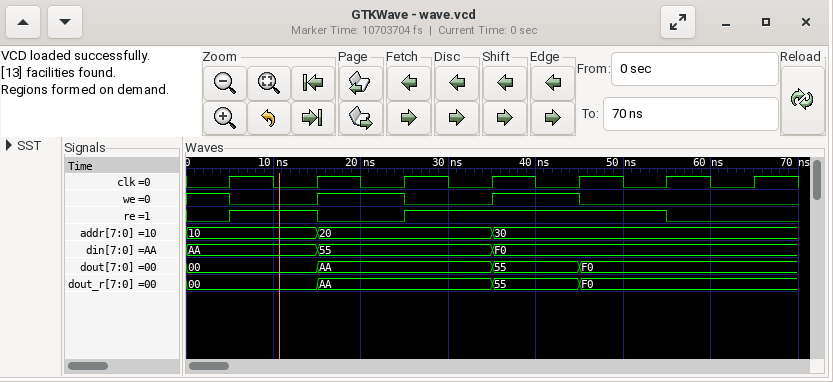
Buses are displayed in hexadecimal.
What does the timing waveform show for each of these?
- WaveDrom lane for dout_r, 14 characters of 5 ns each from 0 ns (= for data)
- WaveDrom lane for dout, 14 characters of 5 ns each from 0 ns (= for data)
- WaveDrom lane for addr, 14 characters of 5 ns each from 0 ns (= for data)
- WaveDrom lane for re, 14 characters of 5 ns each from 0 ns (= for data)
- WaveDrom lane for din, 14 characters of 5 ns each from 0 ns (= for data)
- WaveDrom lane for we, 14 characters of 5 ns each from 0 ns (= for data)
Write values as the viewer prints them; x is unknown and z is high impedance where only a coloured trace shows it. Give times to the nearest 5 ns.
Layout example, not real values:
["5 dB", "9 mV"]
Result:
["{name: 'dout_r', wave: '=..=...=.=....', data: '00 AA 55 F0'}", "{name: 'dout', wave: '=..=...=.=....', data: '00 AA 55 F0'}", "{name: 'addr', wave: '=..=...=......', data: '10 20 30'}", "{name: 're', wave: '01.0.1.....0..'}", "{name: 'din', wave: '=..=...=......', data: 'AA 55 F0'}", "{name: 'we', wave: '10.1.0.1.0....'}"]
